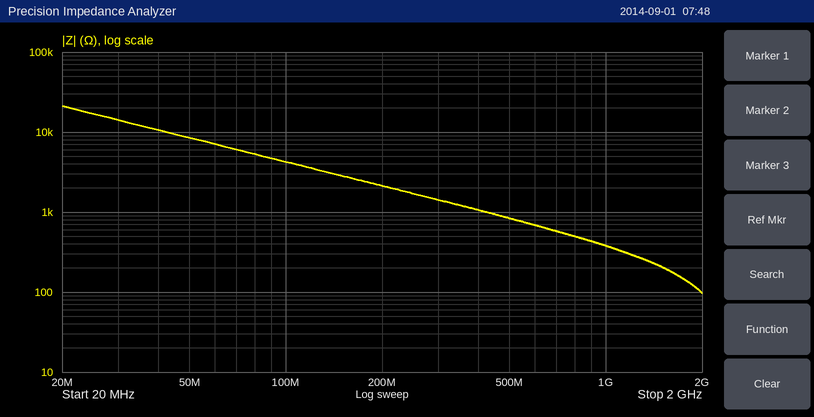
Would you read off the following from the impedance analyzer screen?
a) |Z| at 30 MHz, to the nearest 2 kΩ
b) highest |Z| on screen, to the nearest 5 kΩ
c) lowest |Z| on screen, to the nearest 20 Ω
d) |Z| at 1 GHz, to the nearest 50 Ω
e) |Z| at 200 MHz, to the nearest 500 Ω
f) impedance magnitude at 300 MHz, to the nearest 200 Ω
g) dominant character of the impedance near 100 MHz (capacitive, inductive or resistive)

14 kΩ
20 kΩ
100 Ω
400 Ω
2.0 kΩ
1.4 kΩ
capacitive
